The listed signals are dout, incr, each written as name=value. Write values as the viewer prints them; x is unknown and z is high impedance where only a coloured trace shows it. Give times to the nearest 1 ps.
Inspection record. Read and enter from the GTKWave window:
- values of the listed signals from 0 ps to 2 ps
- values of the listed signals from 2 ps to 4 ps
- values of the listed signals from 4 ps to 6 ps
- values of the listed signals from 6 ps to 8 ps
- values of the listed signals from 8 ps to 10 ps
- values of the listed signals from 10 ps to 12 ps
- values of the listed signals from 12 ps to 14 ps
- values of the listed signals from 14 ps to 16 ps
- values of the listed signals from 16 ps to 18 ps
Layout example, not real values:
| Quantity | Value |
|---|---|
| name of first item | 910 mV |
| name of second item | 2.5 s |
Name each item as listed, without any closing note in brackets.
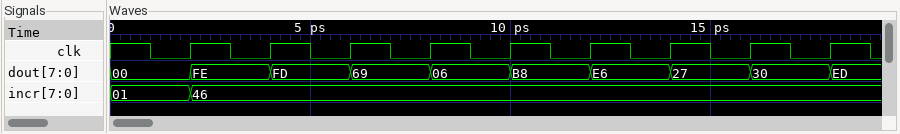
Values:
| Quantity | Value |
|---|---|
| values of the listed signals from 0 ps to 2 ps | dout=00, incr=01 |
| values of the listed signals from 2 ps to 4 ps | dout=FE, incr=46 |
| values of the listed signals from 4 ps to 6 ps | dout=FD, incr=46 |
| values of the listed signals from 6 ps to 8 ps | dout=69, incr=46 |
| values of the listed signals from 8 ps to 10 ps | dout=06, incr=46 |
| values of the listed signals from 10 ps to 12 ps | dout=B8, incr=46 |
| values of the listed signals from 12 ps to 14 ps | dout=E6, incr=46 |
| values of the listed signals from 14 ps to 16 ps | dout=27, incr=46 |
| values of the listed signals from 16 ps to 18 ps | dout=30, incr=46 |
